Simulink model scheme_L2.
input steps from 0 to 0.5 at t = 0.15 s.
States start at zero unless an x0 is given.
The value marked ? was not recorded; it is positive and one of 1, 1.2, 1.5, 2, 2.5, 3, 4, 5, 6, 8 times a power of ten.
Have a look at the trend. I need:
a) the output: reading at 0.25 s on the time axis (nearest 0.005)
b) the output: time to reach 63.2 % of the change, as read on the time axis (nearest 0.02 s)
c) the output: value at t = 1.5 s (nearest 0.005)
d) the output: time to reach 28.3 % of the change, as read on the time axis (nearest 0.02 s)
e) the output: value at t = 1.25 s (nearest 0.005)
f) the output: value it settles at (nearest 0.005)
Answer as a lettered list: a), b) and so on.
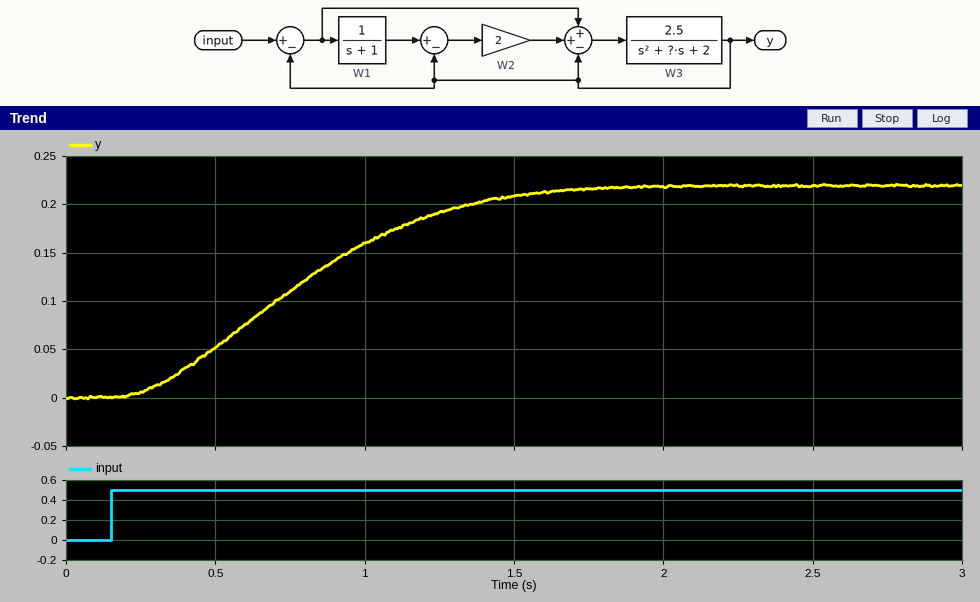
a) 0.005
b) 0.88 s
c) 0.210
d) 0.54 s
e) 0.190
f) 0.220
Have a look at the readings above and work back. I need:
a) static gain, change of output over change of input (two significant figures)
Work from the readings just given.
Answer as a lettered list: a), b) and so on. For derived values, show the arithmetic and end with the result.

a) (0.22 - 0) / (0.5 - 0) = 0.44
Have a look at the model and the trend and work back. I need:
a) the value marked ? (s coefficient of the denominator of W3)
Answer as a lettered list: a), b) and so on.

a) 5
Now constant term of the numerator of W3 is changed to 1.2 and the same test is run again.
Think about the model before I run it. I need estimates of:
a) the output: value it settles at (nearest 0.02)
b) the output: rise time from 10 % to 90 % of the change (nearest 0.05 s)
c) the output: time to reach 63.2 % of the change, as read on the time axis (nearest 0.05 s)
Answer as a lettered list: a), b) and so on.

a) 0.20
b) 1.50 s
c) 1.25 s
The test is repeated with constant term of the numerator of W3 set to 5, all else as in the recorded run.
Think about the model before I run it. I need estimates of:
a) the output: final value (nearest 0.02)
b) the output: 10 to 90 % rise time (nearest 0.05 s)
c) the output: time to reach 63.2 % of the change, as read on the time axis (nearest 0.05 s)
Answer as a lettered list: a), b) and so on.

a) 0.24
b) 0.65 s
c) 0.65 s
